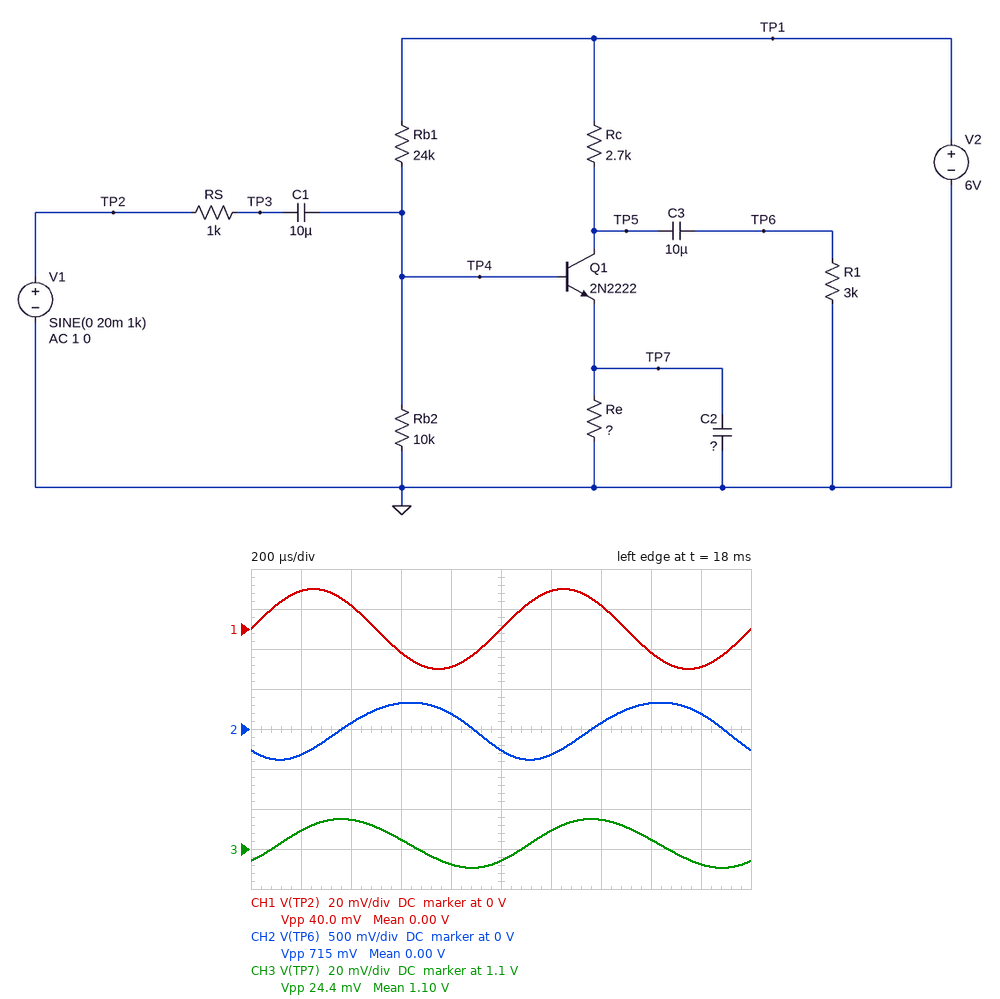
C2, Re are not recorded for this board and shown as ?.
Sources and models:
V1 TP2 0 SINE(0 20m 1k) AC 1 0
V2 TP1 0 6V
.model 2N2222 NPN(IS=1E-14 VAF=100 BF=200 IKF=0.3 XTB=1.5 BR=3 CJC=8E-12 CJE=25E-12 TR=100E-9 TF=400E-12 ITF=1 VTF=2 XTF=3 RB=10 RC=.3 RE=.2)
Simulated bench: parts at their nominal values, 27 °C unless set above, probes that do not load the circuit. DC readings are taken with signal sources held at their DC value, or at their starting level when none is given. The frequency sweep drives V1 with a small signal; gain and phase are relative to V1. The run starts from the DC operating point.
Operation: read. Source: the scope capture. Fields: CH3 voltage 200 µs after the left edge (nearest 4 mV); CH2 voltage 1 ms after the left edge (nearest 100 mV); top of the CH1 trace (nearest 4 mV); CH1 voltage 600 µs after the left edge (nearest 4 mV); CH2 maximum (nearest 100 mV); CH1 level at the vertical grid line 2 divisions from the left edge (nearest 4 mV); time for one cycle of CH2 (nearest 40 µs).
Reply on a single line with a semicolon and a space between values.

1.108 V; -300 mV; 20 mV; -12 mV; 300 mV; 12 mV; 1.00 ms
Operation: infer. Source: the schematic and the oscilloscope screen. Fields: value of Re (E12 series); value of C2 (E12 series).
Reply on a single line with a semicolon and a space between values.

1.8 kΩ; 3.3 µF
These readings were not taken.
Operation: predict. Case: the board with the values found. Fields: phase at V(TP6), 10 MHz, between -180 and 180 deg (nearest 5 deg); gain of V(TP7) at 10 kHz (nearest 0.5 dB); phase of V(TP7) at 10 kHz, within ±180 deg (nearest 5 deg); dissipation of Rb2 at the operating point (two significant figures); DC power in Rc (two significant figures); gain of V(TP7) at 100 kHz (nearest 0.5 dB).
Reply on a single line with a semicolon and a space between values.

90 deg; -21.0 dB; -85 deg; 300 µW; 1.0 mW; -41.0 dB
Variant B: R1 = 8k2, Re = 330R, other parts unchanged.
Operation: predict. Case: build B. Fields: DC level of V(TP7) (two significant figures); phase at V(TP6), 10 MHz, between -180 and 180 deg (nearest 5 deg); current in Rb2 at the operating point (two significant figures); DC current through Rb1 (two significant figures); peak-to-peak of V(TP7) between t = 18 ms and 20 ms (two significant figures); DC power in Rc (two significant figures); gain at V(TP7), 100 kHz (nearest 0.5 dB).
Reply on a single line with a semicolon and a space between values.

660 mV; 65 deg; 130 µA; 190 µA; 2.2 mV; 10 mW; -65.0 dB
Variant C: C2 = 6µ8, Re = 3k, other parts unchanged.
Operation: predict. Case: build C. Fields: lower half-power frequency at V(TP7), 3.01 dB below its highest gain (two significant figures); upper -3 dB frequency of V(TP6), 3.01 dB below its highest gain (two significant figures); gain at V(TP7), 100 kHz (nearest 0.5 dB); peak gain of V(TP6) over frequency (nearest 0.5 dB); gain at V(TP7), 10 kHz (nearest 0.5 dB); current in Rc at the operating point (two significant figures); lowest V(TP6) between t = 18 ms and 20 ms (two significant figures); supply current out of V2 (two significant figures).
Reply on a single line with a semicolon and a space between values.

2.0 Hz; 1.3 MHz; -51.0 dB; 24.5 dB; -31.0 dB; 370 µA; -350 mV; 550 µA
